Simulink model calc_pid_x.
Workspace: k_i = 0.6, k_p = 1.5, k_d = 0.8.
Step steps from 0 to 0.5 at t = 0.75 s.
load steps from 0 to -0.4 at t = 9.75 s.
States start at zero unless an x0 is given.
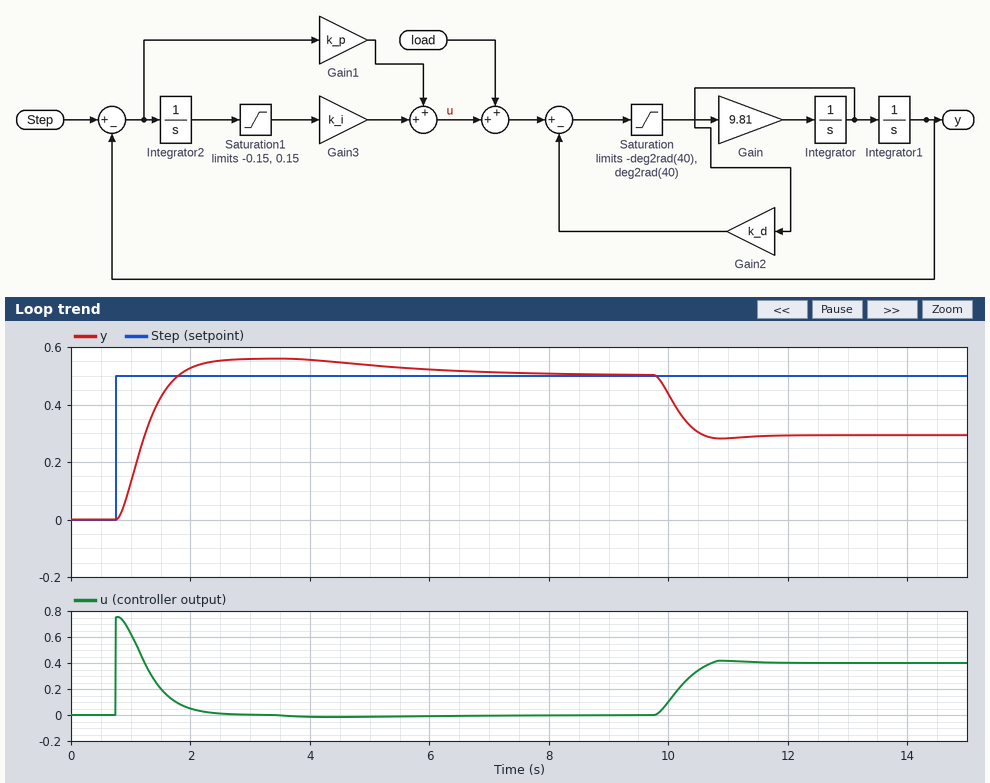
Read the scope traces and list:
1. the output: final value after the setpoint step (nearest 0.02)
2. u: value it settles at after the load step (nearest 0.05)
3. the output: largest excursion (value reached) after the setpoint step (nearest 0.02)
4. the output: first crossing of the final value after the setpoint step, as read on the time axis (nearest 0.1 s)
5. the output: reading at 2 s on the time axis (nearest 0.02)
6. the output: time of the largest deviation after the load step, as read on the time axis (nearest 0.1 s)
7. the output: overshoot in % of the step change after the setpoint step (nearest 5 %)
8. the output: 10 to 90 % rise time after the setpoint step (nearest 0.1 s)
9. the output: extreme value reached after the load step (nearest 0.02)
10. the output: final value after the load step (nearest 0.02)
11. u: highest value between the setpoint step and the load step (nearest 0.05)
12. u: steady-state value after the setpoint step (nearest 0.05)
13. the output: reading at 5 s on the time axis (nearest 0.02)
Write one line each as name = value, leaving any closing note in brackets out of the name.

the output: final value after the setpoint step = 0.50
u: value it settles at after the load step = 0.40
the output: largest excursion (value reached) after the setpoint step = 0.56
the output: first crossing of the final value after the setpoint step, as read on the time axis = 1.8 s
the output: reading at 2 s on the time axis = 0.52
the output: time of the largest deviation after the load step, as read on the time axis = 10.9 s
the output: overshoot in % of the step change after the setpoint step = 10 %
the output: 10 to 90 % rise time after the setpoint step = 0.7 s
the output: extreme value reached after the load step = 0.28
the output: final value after the load step = 0.30
u: highest value between the setpoint step and the load step = 0.75
u: steady-state value after the setpoint step = 0.00
the output: reading at 5 s on the time axis = 0.54
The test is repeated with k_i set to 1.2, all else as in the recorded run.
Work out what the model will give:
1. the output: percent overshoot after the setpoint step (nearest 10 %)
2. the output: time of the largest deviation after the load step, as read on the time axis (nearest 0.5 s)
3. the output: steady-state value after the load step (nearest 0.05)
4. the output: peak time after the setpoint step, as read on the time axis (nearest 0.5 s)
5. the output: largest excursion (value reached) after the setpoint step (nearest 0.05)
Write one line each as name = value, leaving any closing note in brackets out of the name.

the output: percent overshoot after the setpoint step = 20 %
the output: time of the largest deviation after the load step, as read on the time axis = 10.5 s
the output: steady-state value after the load step = 0.35
the output: peak time after the setpoint step, as read on the time axis = 2.5 s
the output: largest excursion (value reached) after the setpoint step = 0.60
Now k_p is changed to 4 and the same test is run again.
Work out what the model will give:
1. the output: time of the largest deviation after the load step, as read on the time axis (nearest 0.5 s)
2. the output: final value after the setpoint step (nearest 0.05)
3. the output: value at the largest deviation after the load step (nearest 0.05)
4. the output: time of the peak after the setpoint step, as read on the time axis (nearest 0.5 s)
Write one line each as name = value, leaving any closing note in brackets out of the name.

the output: time of the largest deviation after the load step, as read on the time axis = 10.5 s
the output: final value after the setpoint step = 0.50
the output: value at the largest deviation after the load step = 0.40
the output: time of the peak after the setpoint step, as read on the time axis = 1.5 s
